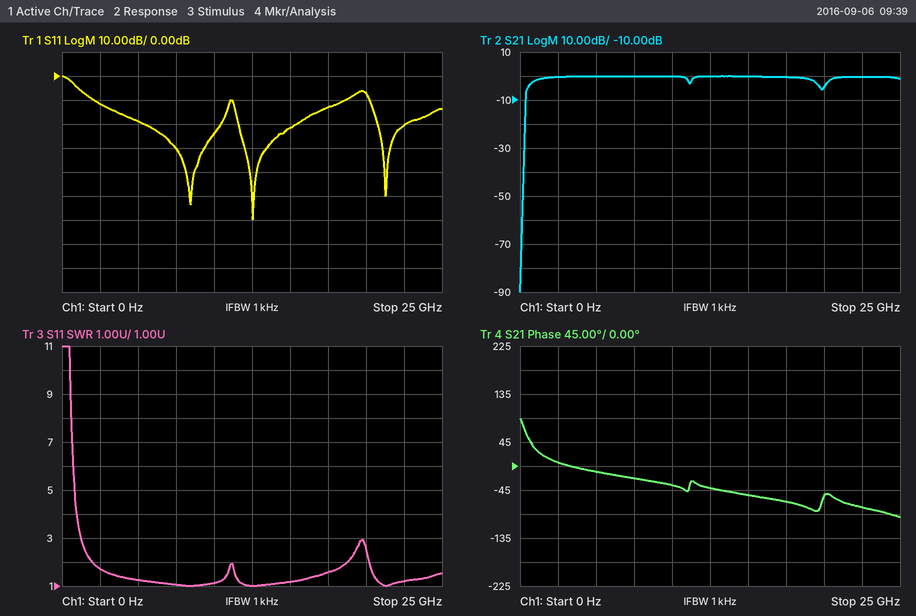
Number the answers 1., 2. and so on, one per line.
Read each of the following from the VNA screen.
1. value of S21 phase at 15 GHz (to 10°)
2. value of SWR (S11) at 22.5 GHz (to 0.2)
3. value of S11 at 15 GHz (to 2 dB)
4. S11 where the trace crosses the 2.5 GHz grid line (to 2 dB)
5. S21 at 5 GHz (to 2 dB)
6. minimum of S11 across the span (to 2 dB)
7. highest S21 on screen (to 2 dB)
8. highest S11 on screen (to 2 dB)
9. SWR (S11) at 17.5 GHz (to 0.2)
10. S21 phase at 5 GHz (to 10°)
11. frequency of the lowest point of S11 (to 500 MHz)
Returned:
1. -50°
2. 1.2
3. -22 dB
4. -12 dB
5. 0 dB
6. -60 dB
7. 0 dB
8. 0 dB
9. 1.6
10. -10°
11. 12.5 GHz
